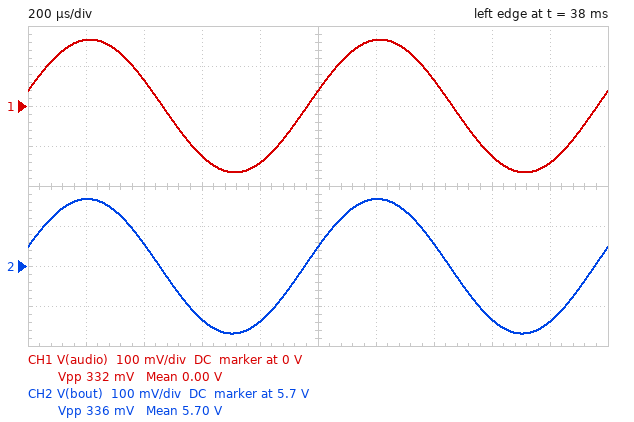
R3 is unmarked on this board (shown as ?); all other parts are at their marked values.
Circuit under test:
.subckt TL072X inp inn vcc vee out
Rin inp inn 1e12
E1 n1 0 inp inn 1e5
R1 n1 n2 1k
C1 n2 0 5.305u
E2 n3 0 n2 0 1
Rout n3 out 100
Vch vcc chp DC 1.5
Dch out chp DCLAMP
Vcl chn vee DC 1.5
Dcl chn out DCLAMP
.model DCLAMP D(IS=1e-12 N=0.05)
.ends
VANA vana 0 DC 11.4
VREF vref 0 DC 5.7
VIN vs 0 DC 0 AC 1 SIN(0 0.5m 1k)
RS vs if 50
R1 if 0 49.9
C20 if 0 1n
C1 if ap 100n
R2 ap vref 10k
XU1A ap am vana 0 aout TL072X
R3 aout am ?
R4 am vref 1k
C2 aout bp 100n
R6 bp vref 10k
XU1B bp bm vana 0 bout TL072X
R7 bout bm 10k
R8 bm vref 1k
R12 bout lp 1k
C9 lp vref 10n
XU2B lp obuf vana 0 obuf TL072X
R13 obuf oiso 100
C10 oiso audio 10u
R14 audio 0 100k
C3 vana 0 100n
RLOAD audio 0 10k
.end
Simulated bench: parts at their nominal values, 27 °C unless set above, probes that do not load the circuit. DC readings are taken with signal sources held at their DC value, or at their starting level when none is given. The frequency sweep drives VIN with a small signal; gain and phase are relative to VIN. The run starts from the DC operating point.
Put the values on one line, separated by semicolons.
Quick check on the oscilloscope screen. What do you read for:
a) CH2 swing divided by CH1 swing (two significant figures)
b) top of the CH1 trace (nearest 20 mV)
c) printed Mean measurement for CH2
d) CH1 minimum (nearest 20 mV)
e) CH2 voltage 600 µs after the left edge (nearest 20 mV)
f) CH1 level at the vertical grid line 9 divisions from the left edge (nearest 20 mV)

1.0; 160 mV; 5.70 V; -160 mV; 5.56 V; -140 mV
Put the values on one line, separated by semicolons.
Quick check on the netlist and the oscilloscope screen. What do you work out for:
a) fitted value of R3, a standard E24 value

62 kΩ
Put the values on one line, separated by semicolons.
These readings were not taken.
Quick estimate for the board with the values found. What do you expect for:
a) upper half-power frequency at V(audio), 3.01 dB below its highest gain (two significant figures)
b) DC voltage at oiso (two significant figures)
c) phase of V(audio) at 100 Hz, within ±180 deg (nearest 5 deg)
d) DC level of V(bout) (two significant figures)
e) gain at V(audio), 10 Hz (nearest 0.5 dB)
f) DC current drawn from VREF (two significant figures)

15 kHz; 5.7 V; 115 deg; 5.7 V; 2.5 dB; 110 nA
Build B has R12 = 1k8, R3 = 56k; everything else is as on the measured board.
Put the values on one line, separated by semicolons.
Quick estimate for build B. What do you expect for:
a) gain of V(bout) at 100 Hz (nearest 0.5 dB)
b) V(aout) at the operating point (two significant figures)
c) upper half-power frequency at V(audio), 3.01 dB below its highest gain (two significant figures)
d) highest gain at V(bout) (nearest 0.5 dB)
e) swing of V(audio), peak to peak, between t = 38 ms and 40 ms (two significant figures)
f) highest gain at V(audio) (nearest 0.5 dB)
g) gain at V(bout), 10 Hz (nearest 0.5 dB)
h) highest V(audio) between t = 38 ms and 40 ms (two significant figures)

39.0 dB; 5.7 V; 9.0 kHz; 50.0 dB; 300 mV; 49.5 dB; 2.0 dB; 150 mV
